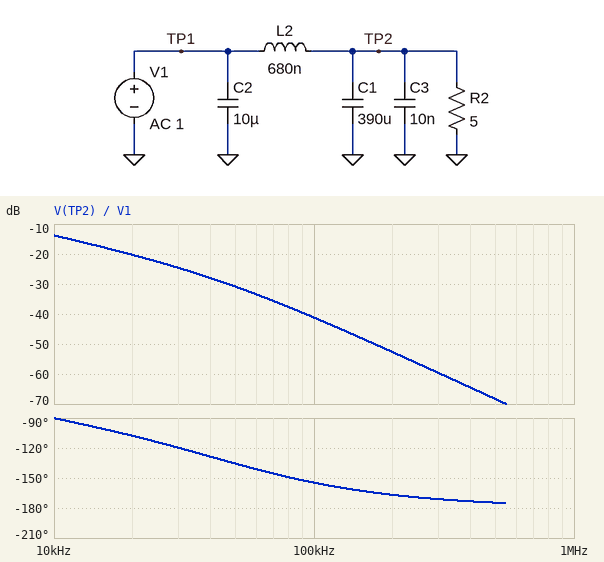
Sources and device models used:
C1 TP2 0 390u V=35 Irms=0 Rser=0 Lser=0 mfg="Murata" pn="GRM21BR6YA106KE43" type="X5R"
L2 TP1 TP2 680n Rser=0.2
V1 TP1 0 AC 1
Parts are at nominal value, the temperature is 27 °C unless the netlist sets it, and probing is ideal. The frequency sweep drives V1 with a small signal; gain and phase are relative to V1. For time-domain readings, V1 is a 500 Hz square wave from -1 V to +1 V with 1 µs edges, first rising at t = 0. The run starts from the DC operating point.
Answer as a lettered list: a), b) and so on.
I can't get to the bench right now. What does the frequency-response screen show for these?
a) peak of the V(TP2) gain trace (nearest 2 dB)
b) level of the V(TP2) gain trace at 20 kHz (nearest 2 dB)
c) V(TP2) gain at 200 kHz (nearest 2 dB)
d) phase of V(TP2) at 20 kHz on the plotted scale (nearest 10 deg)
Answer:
a) -14 dB
b) -20 dB
c) -52 dB
d) -110 deg
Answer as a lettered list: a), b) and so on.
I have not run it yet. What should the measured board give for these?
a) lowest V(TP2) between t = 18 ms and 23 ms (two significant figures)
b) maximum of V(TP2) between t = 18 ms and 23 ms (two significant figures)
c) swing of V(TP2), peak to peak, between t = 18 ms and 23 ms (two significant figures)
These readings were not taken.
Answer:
a) -960 mV
b) 960 mV
c) 1.9 V
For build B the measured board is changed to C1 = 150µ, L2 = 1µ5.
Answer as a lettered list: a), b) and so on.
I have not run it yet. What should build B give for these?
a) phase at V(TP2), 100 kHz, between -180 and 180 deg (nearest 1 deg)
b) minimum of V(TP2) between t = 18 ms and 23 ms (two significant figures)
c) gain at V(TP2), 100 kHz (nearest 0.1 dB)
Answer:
a) -168 deg
b) -960 mV
c) -39.1 dB
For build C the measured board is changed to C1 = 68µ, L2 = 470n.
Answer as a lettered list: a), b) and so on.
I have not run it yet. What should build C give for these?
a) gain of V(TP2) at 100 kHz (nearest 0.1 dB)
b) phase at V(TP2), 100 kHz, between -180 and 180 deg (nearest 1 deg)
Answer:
a) -23.2 dB
b) -143 deg
